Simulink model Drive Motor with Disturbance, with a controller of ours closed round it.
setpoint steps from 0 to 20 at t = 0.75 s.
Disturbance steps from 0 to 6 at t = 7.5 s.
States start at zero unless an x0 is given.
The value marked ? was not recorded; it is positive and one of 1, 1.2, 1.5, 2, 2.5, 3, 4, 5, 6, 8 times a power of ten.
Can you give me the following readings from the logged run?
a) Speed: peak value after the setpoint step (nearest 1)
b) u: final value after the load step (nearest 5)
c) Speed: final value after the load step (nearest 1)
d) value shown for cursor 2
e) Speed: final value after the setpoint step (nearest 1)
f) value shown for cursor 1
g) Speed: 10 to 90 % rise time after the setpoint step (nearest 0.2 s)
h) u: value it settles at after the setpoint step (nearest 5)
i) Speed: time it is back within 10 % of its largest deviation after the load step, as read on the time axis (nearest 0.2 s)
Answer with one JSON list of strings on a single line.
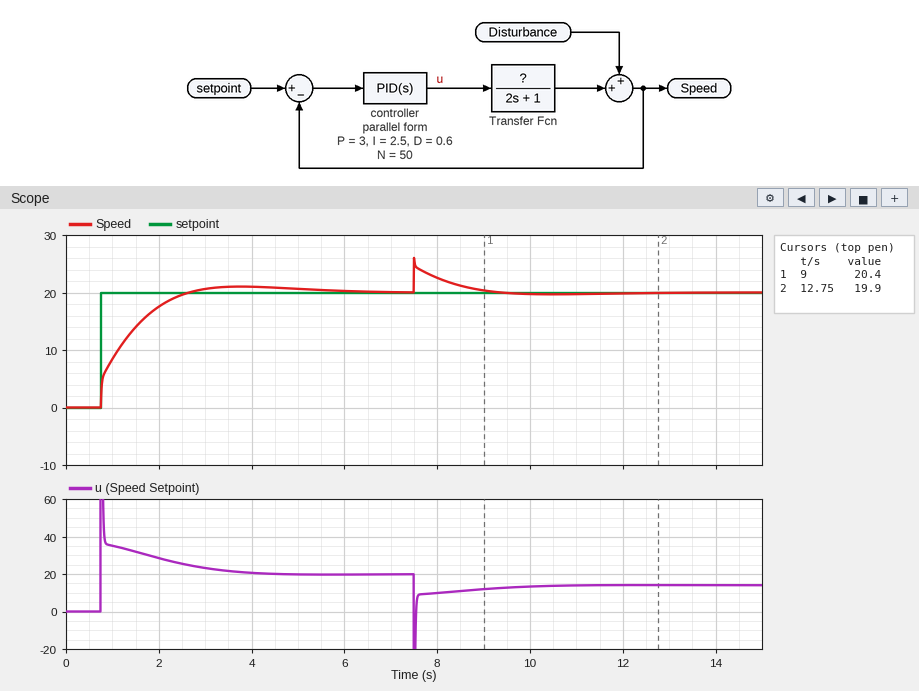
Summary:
["21", "15", "20", "19.9", "20", "20.4", "1.4 s", "20", "8.8 s"]
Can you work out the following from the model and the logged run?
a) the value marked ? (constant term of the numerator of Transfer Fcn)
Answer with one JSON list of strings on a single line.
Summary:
["1"]
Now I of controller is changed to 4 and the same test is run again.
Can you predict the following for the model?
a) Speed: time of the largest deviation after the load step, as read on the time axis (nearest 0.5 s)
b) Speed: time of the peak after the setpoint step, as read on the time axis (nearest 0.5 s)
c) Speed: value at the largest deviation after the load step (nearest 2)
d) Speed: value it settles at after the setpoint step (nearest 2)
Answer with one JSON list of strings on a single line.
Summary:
["7.5 s", "3.0 s", "26", "20"]
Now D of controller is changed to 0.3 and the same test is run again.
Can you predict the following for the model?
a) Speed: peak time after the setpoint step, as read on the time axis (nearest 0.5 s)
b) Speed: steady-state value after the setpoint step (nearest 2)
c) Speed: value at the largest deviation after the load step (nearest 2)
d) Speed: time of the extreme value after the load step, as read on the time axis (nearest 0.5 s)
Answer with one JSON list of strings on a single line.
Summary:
["3.5 s", "20", "26", "7.5 s"]
